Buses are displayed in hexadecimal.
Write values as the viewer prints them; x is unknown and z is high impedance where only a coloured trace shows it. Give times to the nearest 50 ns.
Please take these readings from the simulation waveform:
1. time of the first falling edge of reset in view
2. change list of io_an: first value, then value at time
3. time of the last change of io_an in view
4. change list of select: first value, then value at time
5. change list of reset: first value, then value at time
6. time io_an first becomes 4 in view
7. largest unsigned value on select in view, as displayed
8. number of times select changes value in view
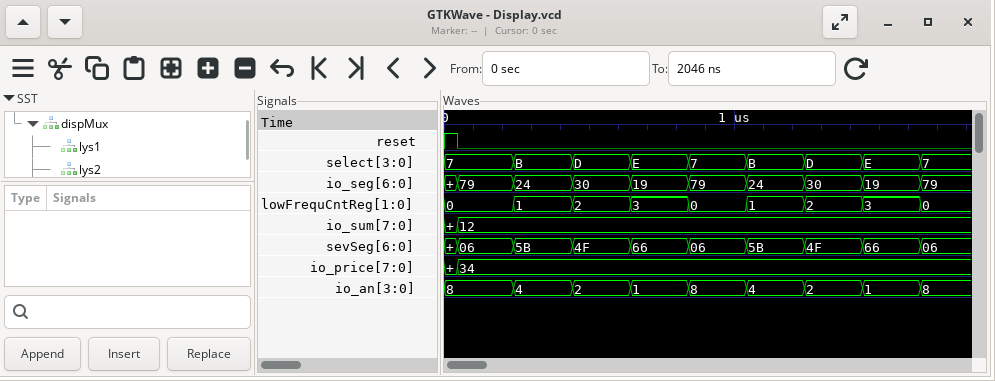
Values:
50 ns
8, 4 at 250 ns, 2 at 450 ns, 1 at 650 ns, 8 at 850 ns, 4 at 1050 ns, 2 at 1250 ns, 1 at 1450 ns, 8 at 1650 ns
1650 ns
7, B at 250 ns, D at 450 ns, E at 650 ns, 7 at 850 ns, B at 1050 ns, D at 1250 ns, E at 1450 ns, 7 at 1650 ns
1, 0 at 50 ns
250 ns
E
8
